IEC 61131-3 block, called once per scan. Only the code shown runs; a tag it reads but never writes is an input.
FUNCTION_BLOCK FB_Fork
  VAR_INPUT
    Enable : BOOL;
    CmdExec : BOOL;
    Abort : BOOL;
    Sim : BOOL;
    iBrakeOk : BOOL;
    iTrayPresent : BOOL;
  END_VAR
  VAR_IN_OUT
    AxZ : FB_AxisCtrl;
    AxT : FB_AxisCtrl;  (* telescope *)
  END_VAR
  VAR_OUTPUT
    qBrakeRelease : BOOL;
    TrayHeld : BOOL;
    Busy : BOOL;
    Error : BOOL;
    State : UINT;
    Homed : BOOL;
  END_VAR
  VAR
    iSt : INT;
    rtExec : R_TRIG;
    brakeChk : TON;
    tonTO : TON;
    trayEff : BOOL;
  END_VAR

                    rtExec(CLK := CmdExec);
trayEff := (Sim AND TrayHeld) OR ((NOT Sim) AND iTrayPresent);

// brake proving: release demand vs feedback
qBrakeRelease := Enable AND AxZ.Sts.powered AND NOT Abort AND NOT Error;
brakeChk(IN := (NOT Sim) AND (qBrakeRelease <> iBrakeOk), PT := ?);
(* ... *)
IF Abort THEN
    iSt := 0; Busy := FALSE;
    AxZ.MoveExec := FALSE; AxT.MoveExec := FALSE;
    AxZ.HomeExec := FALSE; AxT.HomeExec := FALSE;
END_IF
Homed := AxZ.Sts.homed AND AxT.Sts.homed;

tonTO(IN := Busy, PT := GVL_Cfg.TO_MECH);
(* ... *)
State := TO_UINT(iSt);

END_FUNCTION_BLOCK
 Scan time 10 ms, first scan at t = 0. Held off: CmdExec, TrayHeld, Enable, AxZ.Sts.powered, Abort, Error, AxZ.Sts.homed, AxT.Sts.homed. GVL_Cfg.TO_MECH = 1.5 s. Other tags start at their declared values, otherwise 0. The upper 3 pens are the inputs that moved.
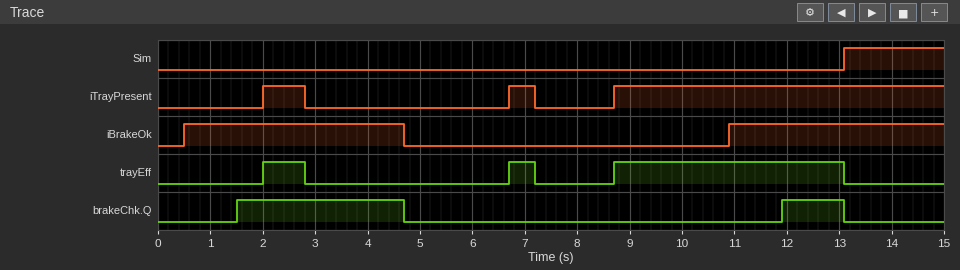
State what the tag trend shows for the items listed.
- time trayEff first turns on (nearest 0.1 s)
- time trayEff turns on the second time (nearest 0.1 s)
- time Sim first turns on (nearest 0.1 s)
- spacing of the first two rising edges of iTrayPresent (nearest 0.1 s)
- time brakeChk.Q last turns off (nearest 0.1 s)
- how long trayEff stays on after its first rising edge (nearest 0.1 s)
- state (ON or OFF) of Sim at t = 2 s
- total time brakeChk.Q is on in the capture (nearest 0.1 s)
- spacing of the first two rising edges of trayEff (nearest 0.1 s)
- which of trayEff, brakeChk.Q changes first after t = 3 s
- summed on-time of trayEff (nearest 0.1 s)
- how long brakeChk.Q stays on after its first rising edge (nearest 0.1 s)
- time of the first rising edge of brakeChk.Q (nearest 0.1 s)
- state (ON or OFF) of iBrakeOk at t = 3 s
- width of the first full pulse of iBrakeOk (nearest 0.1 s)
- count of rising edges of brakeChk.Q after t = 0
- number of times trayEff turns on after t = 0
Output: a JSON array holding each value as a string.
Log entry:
["2.0 s", "6.7 s", "13.1 s", "4.7 s", "13.1 s", "0.8 s", "OFF", "4.4 s", "4.7 s", "brakeChk.Q", "5.7 s", "3.2 s", "1.5 s", "ON", "4.2 s", "2", "3"]
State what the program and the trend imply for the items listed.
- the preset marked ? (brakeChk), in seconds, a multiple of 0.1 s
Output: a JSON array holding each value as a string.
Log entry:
["1.0 s"]
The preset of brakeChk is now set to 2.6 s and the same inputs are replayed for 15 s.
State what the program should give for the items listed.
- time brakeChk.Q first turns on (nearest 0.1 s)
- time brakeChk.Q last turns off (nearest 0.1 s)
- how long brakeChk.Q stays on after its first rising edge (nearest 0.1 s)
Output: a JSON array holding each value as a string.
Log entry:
["3.1 s", "4.7 s", "1.6 s"]
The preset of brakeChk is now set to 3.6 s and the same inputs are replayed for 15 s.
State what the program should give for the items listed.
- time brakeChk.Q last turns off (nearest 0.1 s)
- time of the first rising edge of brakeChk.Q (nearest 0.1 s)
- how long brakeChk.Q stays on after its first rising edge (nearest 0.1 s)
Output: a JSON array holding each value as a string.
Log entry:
["4.7 s", "4.1 s", "0.6 s"]
